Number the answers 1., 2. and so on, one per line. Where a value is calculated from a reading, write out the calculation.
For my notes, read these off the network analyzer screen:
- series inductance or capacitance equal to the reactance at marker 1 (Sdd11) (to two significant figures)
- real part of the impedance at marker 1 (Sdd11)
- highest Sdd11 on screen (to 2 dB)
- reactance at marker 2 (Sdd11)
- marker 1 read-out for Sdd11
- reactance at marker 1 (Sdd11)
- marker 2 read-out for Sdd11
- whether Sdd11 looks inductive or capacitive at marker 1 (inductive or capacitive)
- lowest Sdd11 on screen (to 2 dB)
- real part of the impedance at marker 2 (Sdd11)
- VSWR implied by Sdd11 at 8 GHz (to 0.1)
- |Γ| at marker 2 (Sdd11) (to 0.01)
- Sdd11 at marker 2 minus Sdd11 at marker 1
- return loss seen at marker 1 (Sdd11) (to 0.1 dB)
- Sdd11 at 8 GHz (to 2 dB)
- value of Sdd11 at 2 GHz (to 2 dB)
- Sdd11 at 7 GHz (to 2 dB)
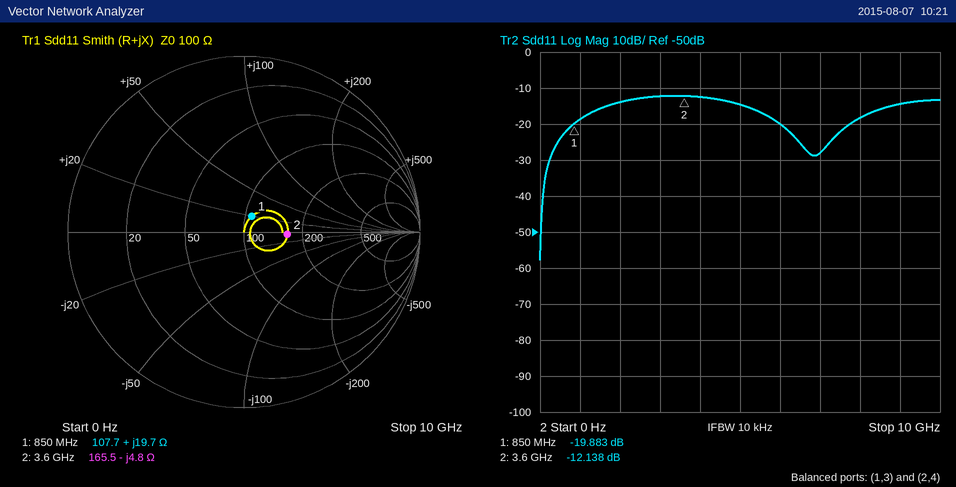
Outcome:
1. L = 19.7 Ω/(2π × 850 MHz) ≈ 3.7 nH
2. 107.7 Ω
3. -12 dB
4. -4.8 Ω
5. -19.883 dB
6. +19.7 Ω
7. -12.138 dB
8. inductive
9. -58 dB
10. 165.5 Ω
11. |Γ| = 10^(-18/20) = 0.1259; VSWR = (1 + 0.1259)/(1 − 0.1259) ≈ 1.3
12. 0.25
13. -12.138 − (-19.883) = 7.745 dB
14. 19.9 dB
15. -18 dB
16. -14 dB
17. -28 dB
